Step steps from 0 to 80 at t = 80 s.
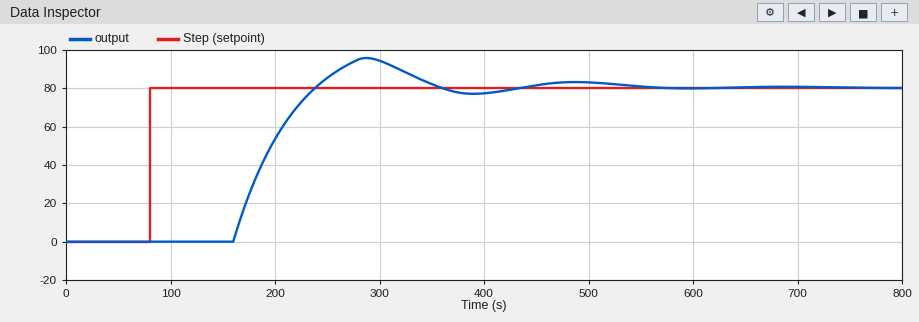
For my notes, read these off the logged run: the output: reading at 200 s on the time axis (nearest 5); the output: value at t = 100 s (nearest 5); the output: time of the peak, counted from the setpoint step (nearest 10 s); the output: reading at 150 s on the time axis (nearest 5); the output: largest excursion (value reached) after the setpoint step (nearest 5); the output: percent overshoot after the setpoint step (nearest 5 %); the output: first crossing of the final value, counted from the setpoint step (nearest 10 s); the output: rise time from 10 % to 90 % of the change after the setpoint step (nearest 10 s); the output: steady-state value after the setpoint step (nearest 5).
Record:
55
0
210 s
0
95
20 %
160 s
60 s
80
